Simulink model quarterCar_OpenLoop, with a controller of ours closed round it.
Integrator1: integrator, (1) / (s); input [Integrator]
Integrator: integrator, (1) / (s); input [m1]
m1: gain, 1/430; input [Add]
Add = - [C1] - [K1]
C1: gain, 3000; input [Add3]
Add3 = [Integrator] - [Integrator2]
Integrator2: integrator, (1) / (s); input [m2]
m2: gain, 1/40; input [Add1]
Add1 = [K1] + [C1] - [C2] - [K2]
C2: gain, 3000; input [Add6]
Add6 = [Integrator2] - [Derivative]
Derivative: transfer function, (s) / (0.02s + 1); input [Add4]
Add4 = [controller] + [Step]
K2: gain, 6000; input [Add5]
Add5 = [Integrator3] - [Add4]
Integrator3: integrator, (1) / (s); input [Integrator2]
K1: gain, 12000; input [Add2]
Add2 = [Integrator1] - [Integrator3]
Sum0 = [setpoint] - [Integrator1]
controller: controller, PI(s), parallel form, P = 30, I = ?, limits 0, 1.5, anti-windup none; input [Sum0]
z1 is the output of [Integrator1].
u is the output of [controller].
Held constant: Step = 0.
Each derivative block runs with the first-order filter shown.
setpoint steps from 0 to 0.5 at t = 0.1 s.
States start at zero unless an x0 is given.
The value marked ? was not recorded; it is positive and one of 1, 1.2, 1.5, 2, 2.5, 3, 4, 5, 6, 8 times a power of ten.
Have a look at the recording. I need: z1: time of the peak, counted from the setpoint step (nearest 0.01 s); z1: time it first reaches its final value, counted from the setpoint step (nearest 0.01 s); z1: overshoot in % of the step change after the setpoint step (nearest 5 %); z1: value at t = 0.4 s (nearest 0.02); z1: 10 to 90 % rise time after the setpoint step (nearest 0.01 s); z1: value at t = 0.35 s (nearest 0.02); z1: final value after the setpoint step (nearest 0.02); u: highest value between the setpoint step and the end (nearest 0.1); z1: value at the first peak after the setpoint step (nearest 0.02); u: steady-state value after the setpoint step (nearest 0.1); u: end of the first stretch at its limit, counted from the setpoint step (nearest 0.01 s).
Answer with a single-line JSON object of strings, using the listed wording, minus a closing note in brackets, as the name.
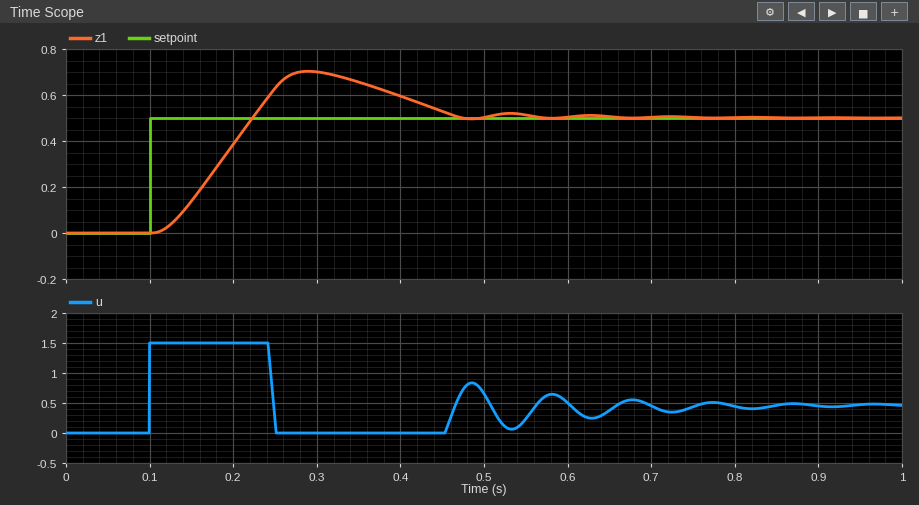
{"z1: time of the peak, counted from the setpoint step": "0.19 s", "z1: time it first reaches its final value, counted from the setpoint step": "0.12 s", "z1: overshoot in % of the step change after the setpoint step": "40 %", "z1: value at t = 0.4 s": "0.60", "z1: 10 to 90 % rise time after the setpoint step": "0.08 s", "z1: value at t = 0.35 s": "0.66", "z1: final value after the setpoint step": "0.50", "u: highest value between the setpoint step and the end": "1.5", "z1: value at the first peak after the setpoint step": "0.70", "u: steady-state value after the setpoint step": "0.5", "u: end of the first stretch at its limit, counted from the setpoint step": "0.14 s"}
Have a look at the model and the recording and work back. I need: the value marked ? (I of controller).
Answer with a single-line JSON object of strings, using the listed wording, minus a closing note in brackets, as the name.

{"the value marked ?": "120"}
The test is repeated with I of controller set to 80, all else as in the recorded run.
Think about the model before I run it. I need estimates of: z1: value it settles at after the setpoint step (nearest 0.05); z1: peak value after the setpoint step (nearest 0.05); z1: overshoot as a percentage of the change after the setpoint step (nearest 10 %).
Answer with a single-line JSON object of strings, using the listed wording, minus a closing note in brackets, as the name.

{"z1: value it settles at after the setpoint step": "0.50", "z1: peak value after the setpoint step": "0.65", "z1: overshoot as a percentage of the change after the setpoint step": "30 %"}
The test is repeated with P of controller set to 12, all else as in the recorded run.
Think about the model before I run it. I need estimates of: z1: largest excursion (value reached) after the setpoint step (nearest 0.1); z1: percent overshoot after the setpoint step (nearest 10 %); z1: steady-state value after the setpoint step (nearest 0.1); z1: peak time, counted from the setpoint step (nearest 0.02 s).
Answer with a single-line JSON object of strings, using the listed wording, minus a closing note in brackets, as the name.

{"z1: largest excursion (value reached) after the setpoint step": "0.8", "z1: percent overshoot after the setpoint step": "60 %", "z1: steady-state value after the setpoint step": "0.5", "z1: peak time, counted from the setpoint step": "0.22 s"}
